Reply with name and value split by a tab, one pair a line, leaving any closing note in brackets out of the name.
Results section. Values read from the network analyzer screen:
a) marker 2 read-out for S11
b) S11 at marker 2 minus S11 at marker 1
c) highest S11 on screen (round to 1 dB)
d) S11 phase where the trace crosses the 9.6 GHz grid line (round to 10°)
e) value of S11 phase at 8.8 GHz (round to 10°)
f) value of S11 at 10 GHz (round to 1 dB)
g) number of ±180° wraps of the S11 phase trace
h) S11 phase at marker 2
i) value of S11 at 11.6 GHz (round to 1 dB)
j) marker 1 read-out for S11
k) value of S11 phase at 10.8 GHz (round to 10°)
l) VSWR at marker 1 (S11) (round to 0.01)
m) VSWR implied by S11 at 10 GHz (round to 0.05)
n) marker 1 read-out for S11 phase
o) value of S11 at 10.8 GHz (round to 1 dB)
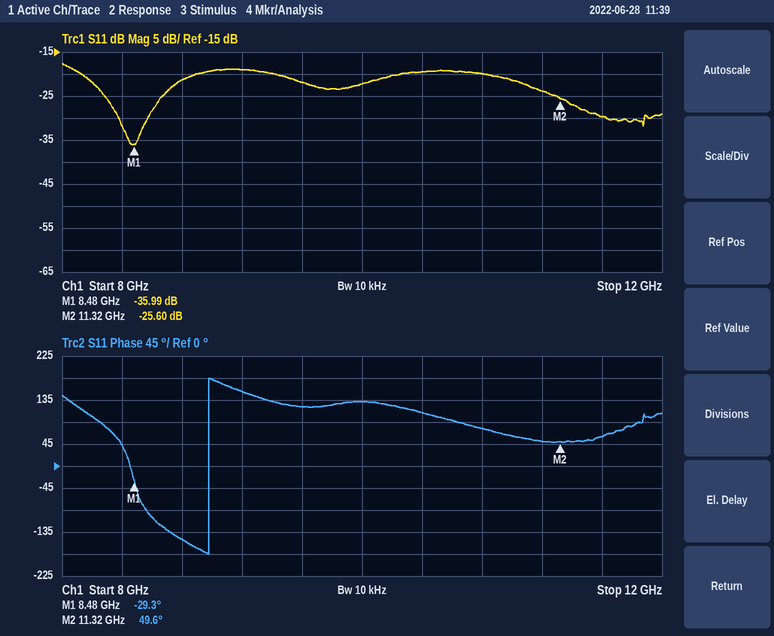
marker 2 read-out for S11	-25.60 dB
S11 at marker 2 minus S11 at marker 1	10.39 dB
highest S11 on screen	-18 dB
S11 phase where the trace crosses the 9.6 GHz grid line	120°
value of S11 phase at 8.8 GHz	-150°
value of S11 at 10 GHz	-22 dB
number of ±180° wraps of the S11 phase trace	1
S11 phase at marker 2	49.6°
value of S11 at 11.6 GHz	-30 dB
marker 1 read-out for S11	-35.99 dB
value of S11 phase at 10.8 GHz	80°
VSWR at marker 1 (S11)	1.03
VSWR implied by S11 at 10 GHz	1.15
marker 1 read-out for S11 phase	-29.3°
value of S11 at 10.8 GHz	-20 dB
